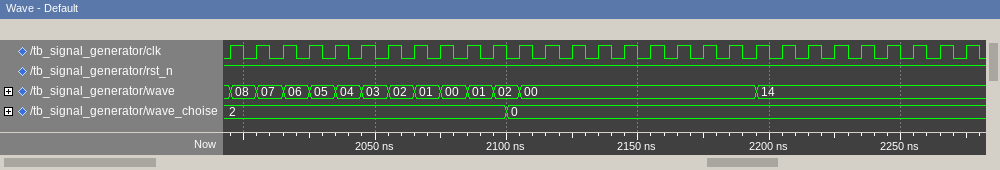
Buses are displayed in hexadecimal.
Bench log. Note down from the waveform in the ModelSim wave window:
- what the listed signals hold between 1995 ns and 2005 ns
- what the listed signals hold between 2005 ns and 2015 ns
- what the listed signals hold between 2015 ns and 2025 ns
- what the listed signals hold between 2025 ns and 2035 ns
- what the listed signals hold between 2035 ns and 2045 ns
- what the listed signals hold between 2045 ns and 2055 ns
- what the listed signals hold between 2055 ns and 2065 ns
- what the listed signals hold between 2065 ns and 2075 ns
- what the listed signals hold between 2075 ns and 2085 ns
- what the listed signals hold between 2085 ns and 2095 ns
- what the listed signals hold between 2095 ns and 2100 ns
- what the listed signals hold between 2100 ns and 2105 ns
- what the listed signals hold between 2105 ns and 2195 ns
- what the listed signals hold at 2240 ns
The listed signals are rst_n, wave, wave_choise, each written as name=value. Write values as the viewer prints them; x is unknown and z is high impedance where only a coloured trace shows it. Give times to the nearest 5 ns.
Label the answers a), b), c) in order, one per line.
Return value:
a) rst_n=1, wave=08, wave_choise=2
b) rst_n=1, wave=07, wave_choise=2
c) rst_n=1, wave=06, wave_choise=2
d) rst_n=1, wave=05, wave_choise=2
e) rst_n=1, wave=04, wave_choise=2
f) rst_n=1, wave=03, wave_choise=2
g) rst_n=1, wave=02, wave_choise=2
h) rst_n=1, wave=01, wave_choise=2
i) rst_n=1, wave=00, wave_choise=2
j) rst_n=1, wave=01, wave_choise=2
k) rst_n=1, wave=02, wave_choise=2
l) rst_n=1, wave=02, wave_choise=0
m) rst_n=1, wave=00, wave_choise=0
n) rst_n=1, wave=14, wave_choise=0
